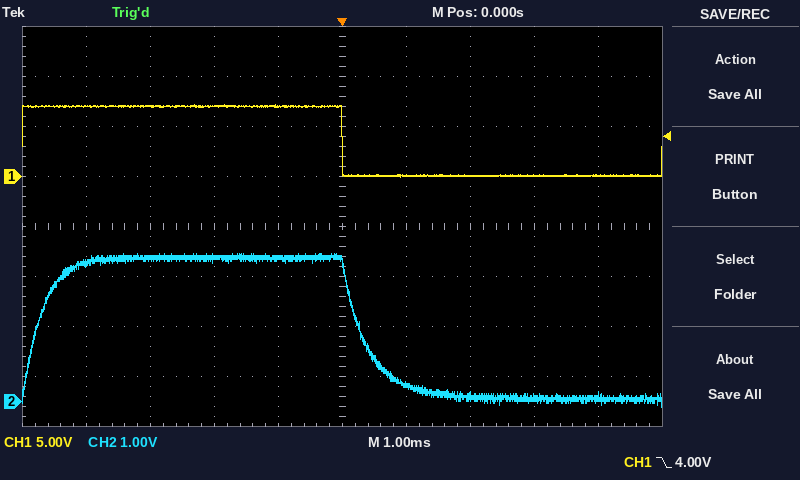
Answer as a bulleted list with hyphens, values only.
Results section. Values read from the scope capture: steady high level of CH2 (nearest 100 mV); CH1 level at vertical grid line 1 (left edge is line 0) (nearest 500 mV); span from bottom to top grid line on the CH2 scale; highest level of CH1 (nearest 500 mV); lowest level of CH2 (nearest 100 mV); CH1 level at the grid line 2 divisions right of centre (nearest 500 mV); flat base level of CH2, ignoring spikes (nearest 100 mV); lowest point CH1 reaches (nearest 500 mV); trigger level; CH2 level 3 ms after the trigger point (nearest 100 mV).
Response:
- 2.9 V
- 7.0 V
- 8 V
- 7.0 V
- -100 mV
- 0.0 V
- 100 mV
- 0.0 V
- 4.00 V
- 100 mV
